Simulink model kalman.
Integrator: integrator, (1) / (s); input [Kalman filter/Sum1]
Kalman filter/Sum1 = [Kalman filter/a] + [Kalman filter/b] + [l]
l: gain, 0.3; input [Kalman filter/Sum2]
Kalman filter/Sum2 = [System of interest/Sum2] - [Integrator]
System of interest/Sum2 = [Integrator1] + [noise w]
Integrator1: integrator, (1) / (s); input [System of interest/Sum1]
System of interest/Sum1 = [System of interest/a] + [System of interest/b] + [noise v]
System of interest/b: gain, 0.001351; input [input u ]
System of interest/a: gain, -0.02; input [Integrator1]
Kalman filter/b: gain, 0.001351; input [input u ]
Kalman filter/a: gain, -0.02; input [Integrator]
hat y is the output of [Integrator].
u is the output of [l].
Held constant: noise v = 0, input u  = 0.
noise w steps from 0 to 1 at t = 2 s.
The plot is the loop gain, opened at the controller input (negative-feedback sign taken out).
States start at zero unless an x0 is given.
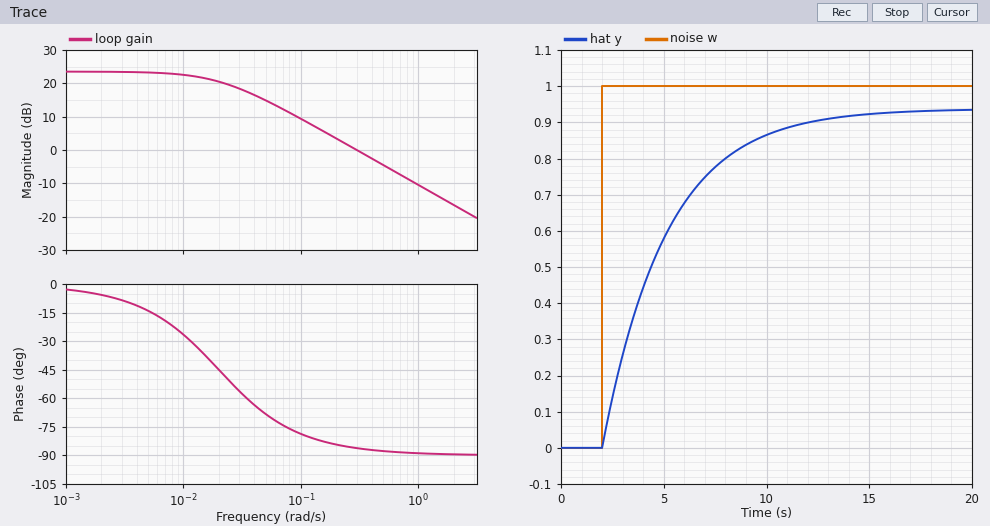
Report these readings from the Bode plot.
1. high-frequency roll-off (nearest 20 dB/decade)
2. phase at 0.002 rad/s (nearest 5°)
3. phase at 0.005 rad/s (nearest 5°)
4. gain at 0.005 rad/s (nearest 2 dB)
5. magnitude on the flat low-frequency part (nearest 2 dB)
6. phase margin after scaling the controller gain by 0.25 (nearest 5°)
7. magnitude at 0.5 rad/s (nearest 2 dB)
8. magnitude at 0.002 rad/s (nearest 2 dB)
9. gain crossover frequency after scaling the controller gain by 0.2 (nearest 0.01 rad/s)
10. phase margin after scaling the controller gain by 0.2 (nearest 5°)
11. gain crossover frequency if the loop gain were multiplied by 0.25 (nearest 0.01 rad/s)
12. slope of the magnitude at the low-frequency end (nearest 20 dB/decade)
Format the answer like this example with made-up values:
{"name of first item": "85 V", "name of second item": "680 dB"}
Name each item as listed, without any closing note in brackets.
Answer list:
{"high-frequency roll-off": "-20 dB/decade", "phase at 0.002 rad/s": "-5°", "phase at 0.005 rad/s": "-15°", "gain at 0.005 rad/s": "24 dB", "magnitude on the flat low-frequency part": "24 dB", "phase margin after scaling the controller gain by 0.25": "105°", "magnitude at 0.5 rad/s": "-4 dB", "magnitude at 0.002 rad/s": "24 dB", "gain crossover frequency after scaling the controller gain by 0.2": "0.06 rad/s", "phase margin after scaling the controller gain by 0.2": "110°", "gain crossover frequency if the loop gain were multiplied by 0.25": "0.07 rad/s", "slope of the magnitude at the low-frequency end": "0 dB/decade"}
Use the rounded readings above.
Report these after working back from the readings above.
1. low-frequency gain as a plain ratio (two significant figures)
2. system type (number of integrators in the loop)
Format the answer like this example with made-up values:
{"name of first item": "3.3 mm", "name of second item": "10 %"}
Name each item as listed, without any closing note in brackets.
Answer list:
{"low-frequency gain as a plain ratio": "16", "system type": "0"}
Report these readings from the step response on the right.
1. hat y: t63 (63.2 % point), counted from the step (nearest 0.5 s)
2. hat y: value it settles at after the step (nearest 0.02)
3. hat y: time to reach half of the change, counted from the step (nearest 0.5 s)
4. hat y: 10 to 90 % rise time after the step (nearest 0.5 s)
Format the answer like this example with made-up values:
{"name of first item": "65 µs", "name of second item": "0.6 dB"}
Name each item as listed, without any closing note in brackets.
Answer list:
{"hat y: t63 (63.2 % point), counted from the step": "3.0 s", "hat y: value it settles at after the step": "0.94", "hat y: time to reach half of the change, counted from the step": "2.0 s", "hat y: 10 to 90 % rise time after the step": "7.0 s"}
